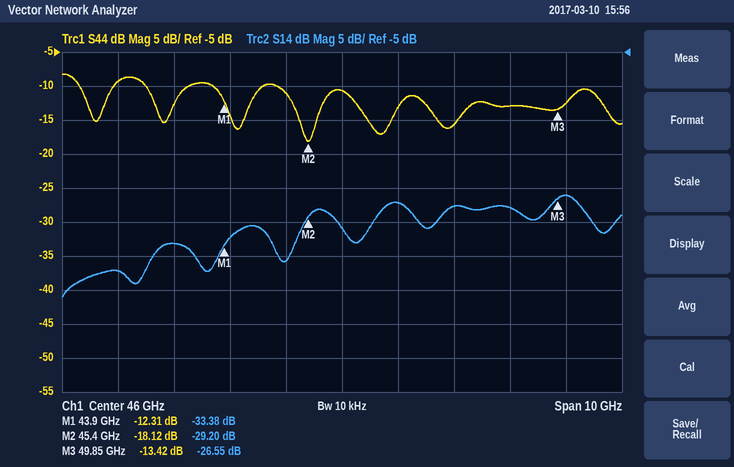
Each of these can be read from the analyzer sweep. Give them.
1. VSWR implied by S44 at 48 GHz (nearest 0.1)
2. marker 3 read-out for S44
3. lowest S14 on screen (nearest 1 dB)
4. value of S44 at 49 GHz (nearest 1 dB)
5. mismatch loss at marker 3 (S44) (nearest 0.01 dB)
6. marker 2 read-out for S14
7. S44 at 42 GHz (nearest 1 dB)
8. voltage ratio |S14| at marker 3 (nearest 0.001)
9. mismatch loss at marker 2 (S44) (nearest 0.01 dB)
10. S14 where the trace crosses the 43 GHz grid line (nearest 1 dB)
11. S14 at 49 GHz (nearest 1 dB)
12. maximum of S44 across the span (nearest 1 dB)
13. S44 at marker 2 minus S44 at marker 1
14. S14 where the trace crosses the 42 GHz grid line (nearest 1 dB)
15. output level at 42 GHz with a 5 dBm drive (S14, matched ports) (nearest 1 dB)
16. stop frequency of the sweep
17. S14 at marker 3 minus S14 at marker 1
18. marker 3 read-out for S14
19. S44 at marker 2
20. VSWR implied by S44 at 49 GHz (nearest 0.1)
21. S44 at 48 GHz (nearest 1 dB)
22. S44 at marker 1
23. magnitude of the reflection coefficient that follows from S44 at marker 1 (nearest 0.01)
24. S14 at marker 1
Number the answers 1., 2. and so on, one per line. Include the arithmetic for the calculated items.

1. |Γ| = 10^(-16/20) = 0.1585; VSWR = (1 + 0.1585)/(1 − 0.1585) ≈ 1.4
2. -13.42 dB
3. -41 dB
4. -13 dB
5. −10 log10(1 − 10^(-13.42/10)) ≈ 0.20 dB
6. -29.20 dB
7. -9 dB
8. 10^(-26.55/20) ≈ 0.047
9. −10 log10(1 − 10^(-18.12/10)) ≈ 0.07 dB
10. -33 dB
11. -28 dB
12. -8 dB
13. -18.12 − (-12.31) = -5.81 dB
14. -37 dB
15. 5 dBm + (-37 dB) = -32 dBm
16. 51 GHz
17. -26.55 − (-33.38) = 6.83 dB
18. -26.55 dB
19. -18.12 dB
20. |Γ| = 10^(-13/20) = 0.2239; VSWR = (1 + 0.2239)/(1 − 0.2239) ≈ 1.6
21. -16 dB
22. -12.31 dB
23. 10^(-12.31/20) ≈ 0.24
24. -33.38 dB
